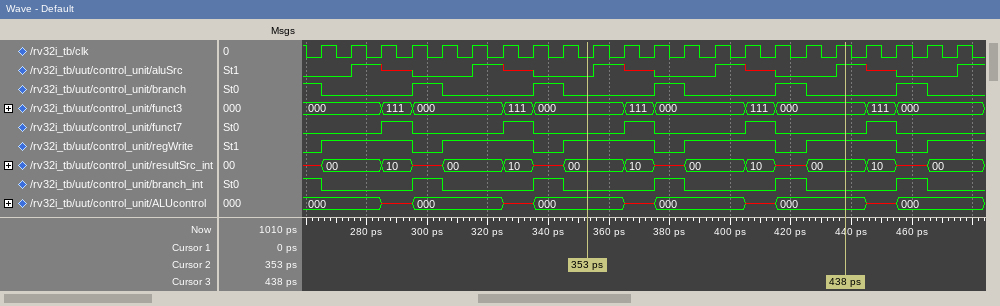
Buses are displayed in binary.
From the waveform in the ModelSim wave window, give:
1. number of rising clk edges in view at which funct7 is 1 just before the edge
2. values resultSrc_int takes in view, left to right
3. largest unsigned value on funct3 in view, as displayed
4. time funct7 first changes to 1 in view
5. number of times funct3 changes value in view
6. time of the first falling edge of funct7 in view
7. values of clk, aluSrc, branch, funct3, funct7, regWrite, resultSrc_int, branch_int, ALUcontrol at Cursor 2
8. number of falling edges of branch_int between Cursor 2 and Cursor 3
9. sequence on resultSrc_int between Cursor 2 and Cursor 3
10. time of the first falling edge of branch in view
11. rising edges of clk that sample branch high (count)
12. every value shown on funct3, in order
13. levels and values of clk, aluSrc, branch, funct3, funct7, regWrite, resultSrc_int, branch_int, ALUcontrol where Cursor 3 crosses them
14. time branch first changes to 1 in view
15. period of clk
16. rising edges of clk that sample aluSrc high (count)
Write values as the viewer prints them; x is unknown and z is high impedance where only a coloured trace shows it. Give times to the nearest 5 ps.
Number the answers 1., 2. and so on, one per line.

1. 5
2. x, 00, 10, x, 00, 10, x, 00, 10, x, 00, 10, x, 00, 10, x, 00
3. 111
4. 285 ps
5. 10
6. 295 ps
7. clk=0, aluSrc=0, branch=0, funct3=000, funct7=0, regWrite=1, resultSrc_int=00, branch_int=0, ALUcontrol=000
8. 2
9. 00, 10, x, 00, 10, x, 00
10. 265 ps
11. 6
12. 000, 111, 000, 111, 000, 111, 000, 111, 000, 111, 000
13. clk=1, aluSrc=1, branch=0, funct3=000, funct7=0, regWrite=1, resultSrc_int=00, branch_int=0, ALUcontrol=000
14. 295 ps
15. 10 ps
16. 5
